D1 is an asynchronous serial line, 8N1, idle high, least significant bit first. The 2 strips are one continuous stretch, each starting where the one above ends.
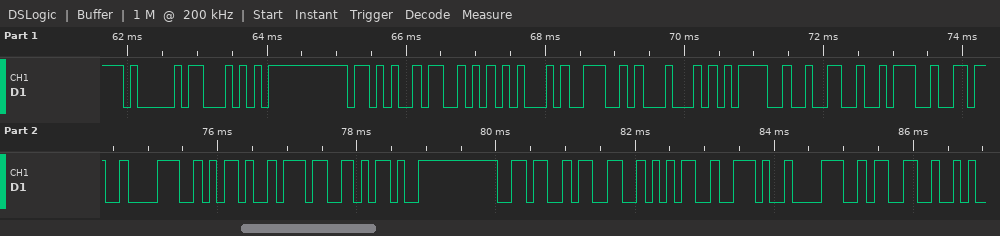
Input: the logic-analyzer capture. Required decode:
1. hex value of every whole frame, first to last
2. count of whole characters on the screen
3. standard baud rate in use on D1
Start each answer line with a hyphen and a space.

- 41 54 2B 53 45 4E 44 3D 32 3A 36 38 2D 37 2D 36 33 35 2E 38 33
- 21
- 9600 baud
